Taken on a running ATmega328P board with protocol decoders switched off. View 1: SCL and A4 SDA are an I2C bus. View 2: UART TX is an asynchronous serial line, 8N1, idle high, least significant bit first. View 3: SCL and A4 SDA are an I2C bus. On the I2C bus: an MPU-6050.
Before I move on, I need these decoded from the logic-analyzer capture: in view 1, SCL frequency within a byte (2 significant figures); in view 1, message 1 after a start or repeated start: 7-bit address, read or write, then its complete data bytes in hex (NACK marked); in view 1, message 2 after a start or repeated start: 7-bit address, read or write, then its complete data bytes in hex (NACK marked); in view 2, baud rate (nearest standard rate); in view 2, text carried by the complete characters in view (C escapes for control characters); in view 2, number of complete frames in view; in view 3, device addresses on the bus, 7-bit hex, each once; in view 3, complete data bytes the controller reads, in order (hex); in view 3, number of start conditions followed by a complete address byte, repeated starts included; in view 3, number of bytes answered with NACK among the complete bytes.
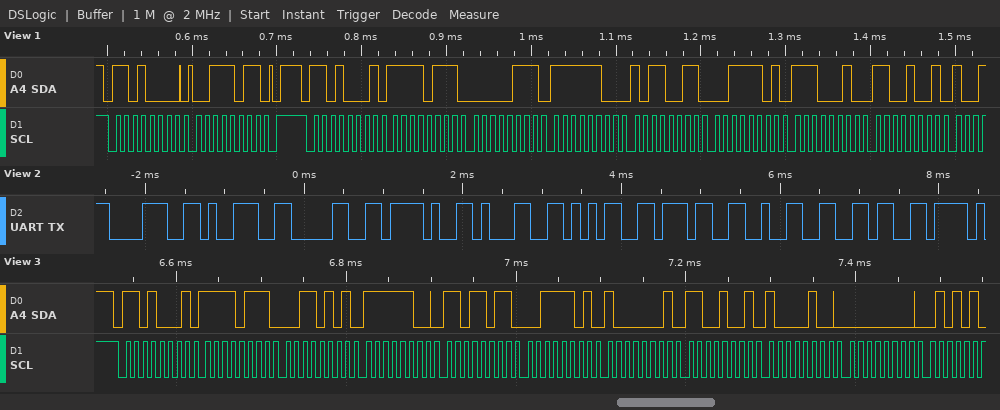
100 kHz
0x68 write: 3B
0x68 read: F7 07 FC B3 3D E2 C9
9600 baud
"890/15726"
9
0x68
F7 35 FC DB 3D 81 C9 84 00
1
0
